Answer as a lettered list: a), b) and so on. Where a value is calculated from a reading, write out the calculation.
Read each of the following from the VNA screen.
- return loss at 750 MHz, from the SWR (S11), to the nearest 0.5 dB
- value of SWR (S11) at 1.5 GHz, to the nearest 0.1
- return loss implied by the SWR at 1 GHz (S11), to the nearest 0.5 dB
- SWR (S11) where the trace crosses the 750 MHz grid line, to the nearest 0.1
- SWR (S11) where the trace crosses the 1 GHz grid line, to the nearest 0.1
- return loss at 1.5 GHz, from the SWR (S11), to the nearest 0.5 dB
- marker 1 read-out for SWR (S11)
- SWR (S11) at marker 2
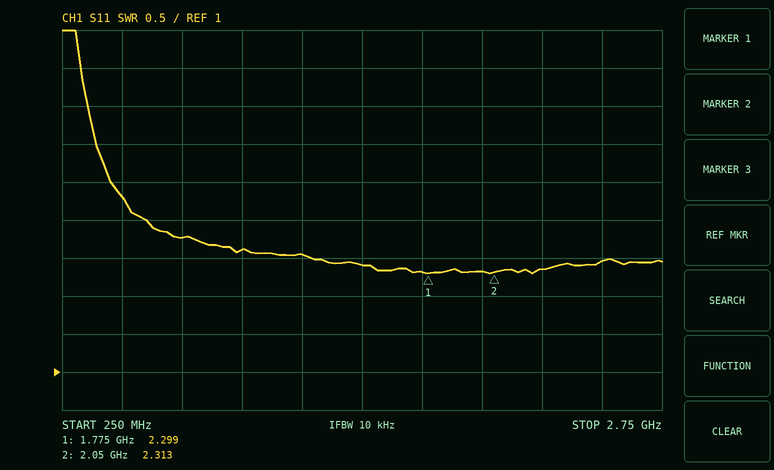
a) −20 log10((2.8 − 1)/(2.8 + 1)) ≈ 6.5 dB
b) 2.4
c) −20 log10((2.6 − 1)/(2.6 + 1)) ≈ 7.0 dB
d) 2.8
e) 2.6
f) −20 log10((2.4 − 1)/(2.4 + 1)) ≈ 7.71 dB, so 7.5 dB to the nearest 0.5 dB
g) 2.299
h) 2.313
